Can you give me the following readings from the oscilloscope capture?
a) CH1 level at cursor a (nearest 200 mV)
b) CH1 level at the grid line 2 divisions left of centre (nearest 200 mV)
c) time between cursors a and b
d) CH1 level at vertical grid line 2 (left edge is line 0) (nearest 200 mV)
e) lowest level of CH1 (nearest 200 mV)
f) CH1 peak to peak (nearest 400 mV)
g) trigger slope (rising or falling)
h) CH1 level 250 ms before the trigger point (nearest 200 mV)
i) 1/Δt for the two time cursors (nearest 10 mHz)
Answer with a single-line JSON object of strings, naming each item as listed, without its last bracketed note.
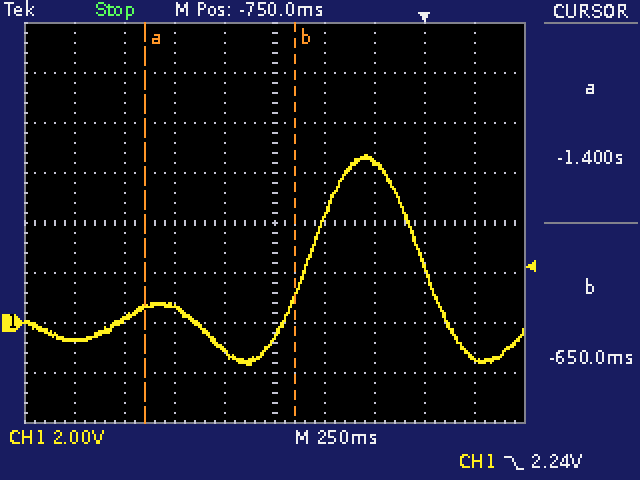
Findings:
{"CH1 level at cursor a": "600 mV", "CH1 level at the grid line 2 divisions left of centre": "600 mV", "time between cursors a and b": "750 ms", "CH1 level at vertical grid line 2 (left edge is line 0)": "200 mV", "lowest level of CH1": "-1.6 V", "CH1 peak to peak": "8.4 V", "trigger slope": "falling", "CH1 level 250 ms before the trigger point": "6.4 V", "1/Δt for the two time cursors": "1.33 Hz"}
